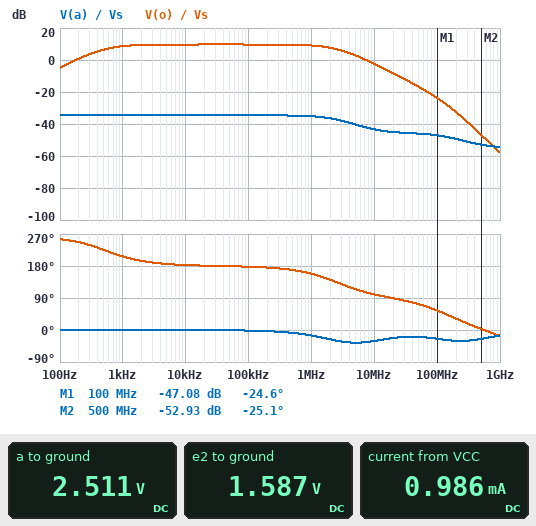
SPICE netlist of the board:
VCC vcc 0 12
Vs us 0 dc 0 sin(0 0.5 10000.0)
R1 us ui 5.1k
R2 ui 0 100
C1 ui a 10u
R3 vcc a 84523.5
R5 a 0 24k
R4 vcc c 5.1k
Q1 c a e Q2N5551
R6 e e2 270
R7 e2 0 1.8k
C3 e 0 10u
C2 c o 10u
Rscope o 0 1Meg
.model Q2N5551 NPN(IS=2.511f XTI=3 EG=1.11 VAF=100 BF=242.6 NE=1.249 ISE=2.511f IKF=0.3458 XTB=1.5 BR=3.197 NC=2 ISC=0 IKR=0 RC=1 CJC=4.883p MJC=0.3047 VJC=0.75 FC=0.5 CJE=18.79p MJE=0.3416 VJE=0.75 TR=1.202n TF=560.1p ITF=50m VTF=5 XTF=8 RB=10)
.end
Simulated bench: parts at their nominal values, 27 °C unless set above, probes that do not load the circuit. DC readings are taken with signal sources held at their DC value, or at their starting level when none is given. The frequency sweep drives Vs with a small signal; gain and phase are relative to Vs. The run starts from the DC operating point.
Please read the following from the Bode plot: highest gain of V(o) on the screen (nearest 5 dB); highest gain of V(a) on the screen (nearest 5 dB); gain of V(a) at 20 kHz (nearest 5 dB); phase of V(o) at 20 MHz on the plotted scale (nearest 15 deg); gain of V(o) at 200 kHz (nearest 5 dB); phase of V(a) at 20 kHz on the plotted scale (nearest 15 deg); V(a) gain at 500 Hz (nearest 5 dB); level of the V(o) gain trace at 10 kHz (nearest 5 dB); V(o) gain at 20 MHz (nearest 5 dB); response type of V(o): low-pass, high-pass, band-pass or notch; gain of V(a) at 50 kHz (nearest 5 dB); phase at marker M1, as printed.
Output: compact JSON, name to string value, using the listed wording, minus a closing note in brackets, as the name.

{"highest gain of V(o) on the screen": "10 dB", "highest gain of V(a) on the screen": "-35 dB", "gain of V(a) at 20 kHz": "-35 dB", "phase of V(o) at 20 MHz on the plotted scale": "90 deg", "gain of V(o) at 200 kHz": "10 dB", "phase of V(a) at 20 kHz on the plotted scale": "0 deg", "V(a) gain at 500 Hz": "-35 dB", "level of the V(o) gain trace at 10 kHz": "10 dB", "V(o) gain at 20 MHz": "-10 dB", "response type of V(o): low-pass, high-pass, band-pass or notch": "band-pass", "gain of V(a) at 50 kHz": "-35 dB", "phase at marker M1, as printed": "-24.6 deg"}
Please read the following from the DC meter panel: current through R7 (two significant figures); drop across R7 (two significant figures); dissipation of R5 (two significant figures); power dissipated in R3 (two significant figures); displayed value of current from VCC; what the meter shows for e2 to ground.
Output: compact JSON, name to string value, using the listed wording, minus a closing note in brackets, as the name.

{"current through R7": "880 µA", "drop across R7": "1.6 V", "dissipation of R5": "260 µW", "power dissipated in R3": "1.1 mW", "displayed value of current from VCC": "0.986 mA", "what the meter shows for e2 to ground": "1.587 V"}
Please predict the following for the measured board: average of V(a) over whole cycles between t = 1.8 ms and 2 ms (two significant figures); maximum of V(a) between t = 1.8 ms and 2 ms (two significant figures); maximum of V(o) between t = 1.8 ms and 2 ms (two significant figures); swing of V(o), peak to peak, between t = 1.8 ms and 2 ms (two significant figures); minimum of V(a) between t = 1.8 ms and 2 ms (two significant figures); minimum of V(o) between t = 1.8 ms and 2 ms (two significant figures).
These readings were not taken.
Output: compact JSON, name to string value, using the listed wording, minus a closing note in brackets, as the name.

{"average of V(a) over whole cycles between t = 1.8 ms and 2 ms": "2.5 V", "maximum of V(a) between t = 1.8 ms and 2 ms": "2.5 V", "maximum of V(o) between t = 1.8 ms and 2 ms": "1.4 V", "swing of V(o), peak to peak, between t = 1.8 ms and 2 ms": "3.0 V", "minimum of V(a) between t = 1.8 ms and 2 ms": "2.5 V", "minimum of V(o) between t = 1.8 ms and 2 ms": "-1.6 V"}
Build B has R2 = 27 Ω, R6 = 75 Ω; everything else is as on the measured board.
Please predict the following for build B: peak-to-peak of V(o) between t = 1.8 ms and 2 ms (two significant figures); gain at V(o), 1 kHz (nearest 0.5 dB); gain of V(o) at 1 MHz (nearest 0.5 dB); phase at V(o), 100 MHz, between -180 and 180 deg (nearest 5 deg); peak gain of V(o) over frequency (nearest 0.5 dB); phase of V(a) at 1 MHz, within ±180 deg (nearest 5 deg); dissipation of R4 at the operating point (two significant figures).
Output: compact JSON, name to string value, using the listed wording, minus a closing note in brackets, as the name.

{"peak-to-peak of V(o) between t = 1.8 ms and 2 ms": "930 mV", "gain at V(o), 1 kHz": "-2.0 dB", "gain of V(o) at 1 MHz": "-1.0 dB", "phase at V(o), 100 MHz, between -180 and 180 deg": "65 deg", "peak gain of V(o) over frequency": "-0.5 dB", "phase of V(a) at 1 MHz, within ±180 deg": "-5 deg", "dissipation of R4 at the operating point": "4.7 mW"}
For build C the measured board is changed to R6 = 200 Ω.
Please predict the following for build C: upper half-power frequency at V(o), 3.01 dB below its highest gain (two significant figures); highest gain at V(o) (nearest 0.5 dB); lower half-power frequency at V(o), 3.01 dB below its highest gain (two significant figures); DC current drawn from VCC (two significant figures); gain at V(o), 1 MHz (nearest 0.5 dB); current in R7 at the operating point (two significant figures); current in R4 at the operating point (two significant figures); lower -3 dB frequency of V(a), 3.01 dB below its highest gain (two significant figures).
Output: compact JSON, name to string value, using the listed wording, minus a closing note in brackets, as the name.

{"upper half-power frequency at V(o), 3.01 dB below its highest gain": "2.5 MHz", "highest gain at V(o)": "10.0 dB", "lower half-power frequency at V(o), 3.01 dB below its highest gain": "530 Hz", "DC current drawn from VCC": "1.0 mA", "gain at V(o), 1 MHz": "9.5 dB", "current in R7 at the operating point": "910 µA", "current in R4 at the operating point": "900 µA", "lower -3 dB frequency of V(a), 3.01 dB below its highest gain": "900 mHz"}
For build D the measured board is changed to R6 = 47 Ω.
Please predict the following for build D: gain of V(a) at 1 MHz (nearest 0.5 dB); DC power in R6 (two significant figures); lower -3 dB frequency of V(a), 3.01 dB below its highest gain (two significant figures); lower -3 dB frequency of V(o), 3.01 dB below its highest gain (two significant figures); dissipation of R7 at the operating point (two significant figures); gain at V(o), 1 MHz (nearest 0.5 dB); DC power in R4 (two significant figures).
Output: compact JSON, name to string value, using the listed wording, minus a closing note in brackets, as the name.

{"gain of V(a) at 1 MHz": "-35.5 dB", "DC power in R6": "45 µW", "lower -3 dB frequency of V(a), 3.01 dB below its highest gain": "910 mHz", "lower -3 dB frequency of V(o), 3.01 dB below its highest gain": "570 Hz", "dissipation of R7 at the operating point": "1.7 mW", "gain at V(o), 1 MHz": "10.0 dB", "DC power in R4": "4.8 mW"}
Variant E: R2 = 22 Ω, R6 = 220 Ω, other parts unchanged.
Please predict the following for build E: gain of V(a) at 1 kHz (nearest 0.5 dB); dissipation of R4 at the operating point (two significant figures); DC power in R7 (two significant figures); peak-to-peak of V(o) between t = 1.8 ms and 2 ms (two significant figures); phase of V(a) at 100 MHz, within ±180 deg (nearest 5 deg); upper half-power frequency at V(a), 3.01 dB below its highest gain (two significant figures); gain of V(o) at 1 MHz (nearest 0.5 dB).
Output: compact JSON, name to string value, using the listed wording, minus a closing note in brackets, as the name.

{"gain of V(a) at 1 kHz": "-47.5 dB", "dissipation of R4 at the operating point": "4.1 mW", "DC power in R7": "1.5 mW", "peak-to-peak of V(o) between t = 1.8 ms and 2 ms": "710 mV", "phase of V(a) at 100 MHz, within ±180 deg": "-15 deg", "upper half-power frequency at V(a), 3.01 dB below its highest gain": "12 MHz", "gain of V(o) at 1 MHz": "-3.0 dB"}
